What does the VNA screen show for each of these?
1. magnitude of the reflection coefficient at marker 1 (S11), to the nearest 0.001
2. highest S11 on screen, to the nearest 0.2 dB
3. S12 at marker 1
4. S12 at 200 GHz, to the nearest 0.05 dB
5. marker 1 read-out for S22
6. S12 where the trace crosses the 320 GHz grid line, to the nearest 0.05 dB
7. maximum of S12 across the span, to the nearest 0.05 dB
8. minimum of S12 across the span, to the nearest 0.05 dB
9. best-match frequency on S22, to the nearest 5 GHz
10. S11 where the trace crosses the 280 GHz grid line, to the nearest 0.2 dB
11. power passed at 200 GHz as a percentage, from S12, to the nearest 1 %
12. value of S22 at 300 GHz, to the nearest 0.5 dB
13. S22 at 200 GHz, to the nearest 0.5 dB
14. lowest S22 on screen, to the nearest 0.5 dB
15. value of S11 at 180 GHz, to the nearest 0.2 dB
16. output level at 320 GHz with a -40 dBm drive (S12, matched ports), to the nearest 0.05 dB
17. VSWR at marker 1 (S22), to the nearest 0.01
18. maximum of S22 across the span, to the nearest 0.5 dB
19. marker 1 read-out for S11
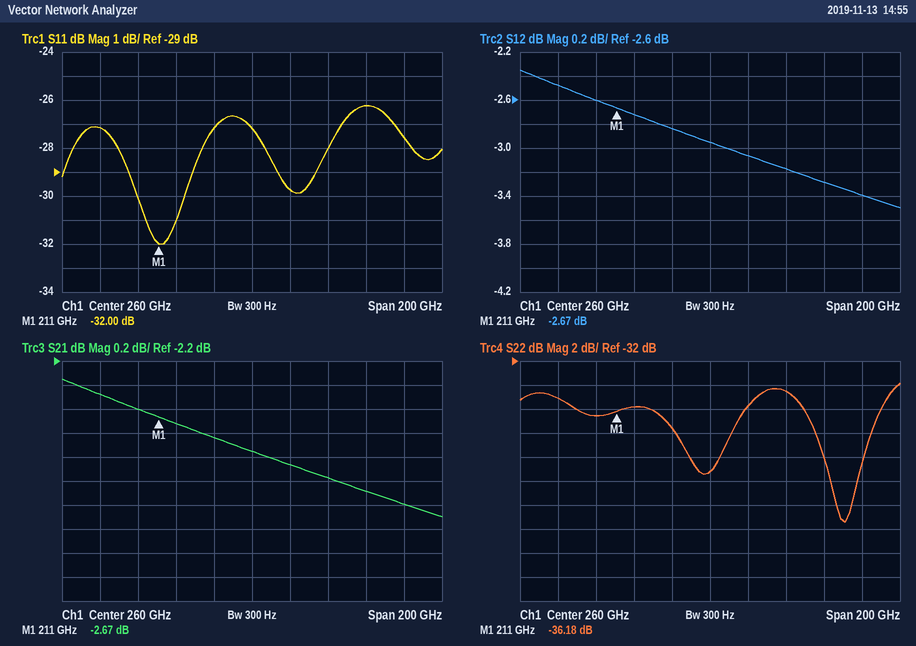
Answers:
0.025
-26.2 dB
-2.67 dB
-2.60 dB
-36.18 dB
-3.30 dB
-2.35 dB
-3.50 dB
330 GHz
-29.8 dB
55 %
-34.5 dB
-36.5 dB
-45.5 dB
-27.2 dB
-43.30 dBm
1.03
-34.0 dB
-32.00 dB
